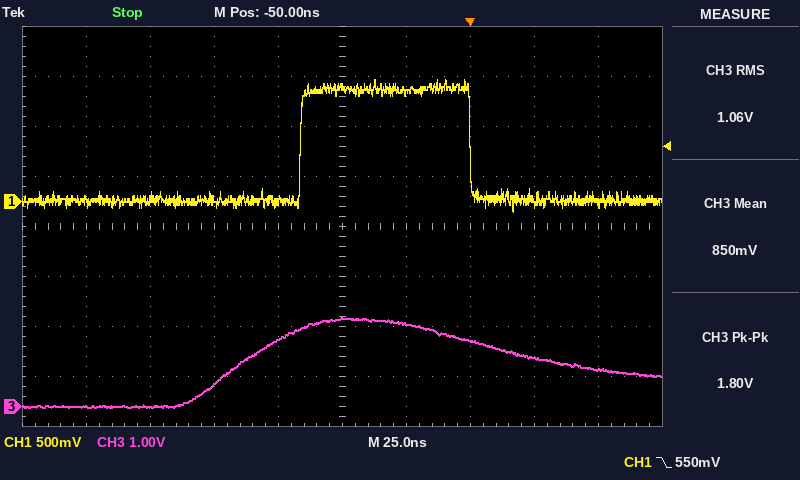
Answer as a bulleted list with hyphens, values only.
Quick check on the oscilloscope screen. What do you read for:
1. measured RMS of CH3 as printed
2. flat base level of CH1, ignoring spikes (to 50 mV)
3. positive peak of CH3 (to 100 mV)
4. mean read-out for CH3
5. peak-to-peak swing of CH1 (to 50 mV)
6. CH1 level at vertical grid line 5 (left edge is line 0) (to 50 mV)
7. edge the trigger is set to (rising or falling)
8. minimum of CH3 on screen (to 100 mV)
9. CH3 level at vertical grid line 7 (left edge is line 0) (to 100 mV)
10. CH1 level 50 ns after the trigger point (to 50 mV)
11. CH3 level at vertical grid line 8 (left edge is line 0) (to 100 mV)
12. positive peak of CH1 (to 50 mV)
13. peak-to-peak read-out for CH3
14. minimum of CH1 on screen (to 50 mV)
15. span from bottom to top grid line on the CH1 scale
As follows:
- 1.06 V
- 0 mV
- 1.8 V
- 850 mV
- 1.30 V
- 1.15 V
- falling
- 0.0 V
- 1.3 V
- 0 mV
- 1.0 V
- 1.20 V
- 1.80 V
- -100 mV
- 4 V
